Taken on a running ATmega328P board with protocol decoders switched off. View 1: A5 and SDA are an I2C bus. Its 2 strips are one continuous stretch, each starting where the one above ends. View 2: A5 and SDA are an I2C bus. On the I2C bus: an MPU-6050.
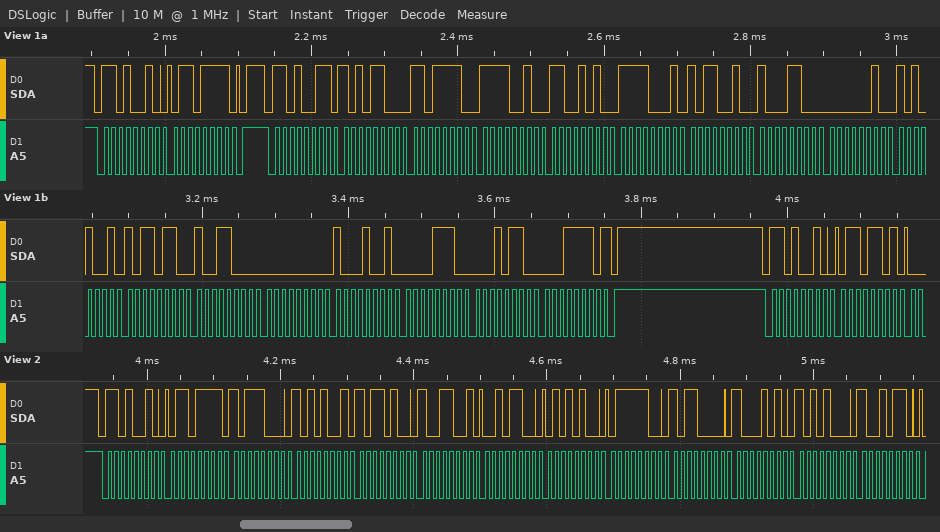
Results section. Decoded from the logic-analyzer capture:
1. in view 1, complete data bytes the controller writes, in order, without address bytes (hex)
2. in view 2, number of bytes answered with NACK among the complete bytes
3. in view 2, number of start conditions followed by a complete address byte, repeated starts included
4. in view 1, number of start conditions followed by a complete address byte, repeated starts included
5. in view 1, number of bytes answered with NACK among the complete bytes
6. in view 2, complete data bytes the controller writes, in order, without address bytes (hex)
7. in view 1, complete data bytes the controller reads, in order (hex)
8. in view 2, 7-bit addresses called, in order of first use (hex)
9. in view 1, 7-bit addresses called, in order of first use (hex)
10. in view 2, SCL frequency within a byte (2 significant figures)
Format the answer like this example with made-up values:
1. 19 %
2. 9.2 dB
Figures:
1. 6F 6D
2. 0
3. 1
4. 3
5. 1
6. 6F B8 A9 B4 99 2C 54 7C B0 8A A8 96
7. AC DE F2 CA F1 B2 8C 02 A9 B6 98 00 89 0E 16 1E
8. 0x69
9. 0x69
10. 100 kHz
